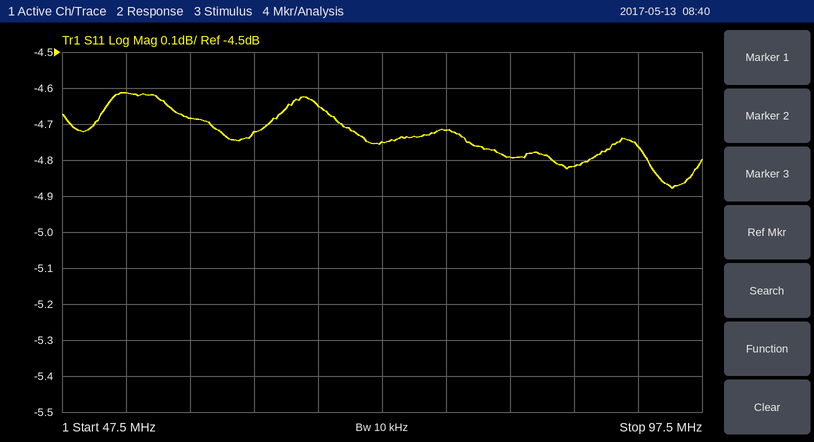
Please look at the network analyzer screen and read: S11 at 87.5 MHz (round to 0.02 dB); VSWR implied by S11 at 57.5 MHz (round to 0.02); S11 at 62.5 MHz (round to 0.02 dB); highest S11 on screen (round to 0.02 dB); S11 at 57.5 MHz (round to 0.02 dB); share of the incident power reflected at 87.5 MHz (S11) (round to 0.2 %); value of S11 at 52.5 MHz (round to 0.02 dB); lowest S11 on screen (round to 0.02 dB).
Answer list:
-4.82 dB
3.80
-4.72 dB
-4.62 dB
-4.68 dB
33.0 %
-4.62 dB
-4.88 dB
